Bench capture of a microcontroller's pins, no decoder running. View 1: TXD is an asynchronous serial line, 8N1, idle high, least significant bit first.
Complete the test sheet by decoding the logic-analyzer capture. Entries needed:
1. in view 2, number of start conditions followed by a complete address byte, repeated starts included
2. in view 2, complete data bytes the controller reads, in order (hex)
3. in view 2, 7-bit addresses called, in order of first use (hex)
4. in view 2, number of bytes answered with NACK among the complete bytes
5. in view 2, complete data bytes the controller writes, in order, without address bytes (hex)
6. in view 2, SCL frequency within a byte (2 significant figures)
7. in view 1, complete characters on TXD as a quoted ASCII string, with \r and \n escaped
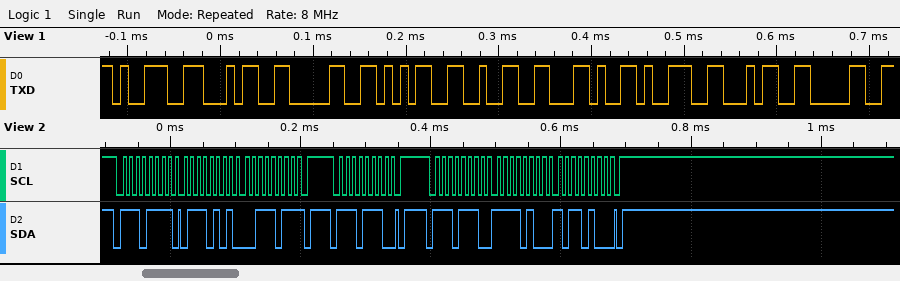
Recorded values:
3
75 3B
0x77
1
F4 B4
100 kHz
"94052,940"
